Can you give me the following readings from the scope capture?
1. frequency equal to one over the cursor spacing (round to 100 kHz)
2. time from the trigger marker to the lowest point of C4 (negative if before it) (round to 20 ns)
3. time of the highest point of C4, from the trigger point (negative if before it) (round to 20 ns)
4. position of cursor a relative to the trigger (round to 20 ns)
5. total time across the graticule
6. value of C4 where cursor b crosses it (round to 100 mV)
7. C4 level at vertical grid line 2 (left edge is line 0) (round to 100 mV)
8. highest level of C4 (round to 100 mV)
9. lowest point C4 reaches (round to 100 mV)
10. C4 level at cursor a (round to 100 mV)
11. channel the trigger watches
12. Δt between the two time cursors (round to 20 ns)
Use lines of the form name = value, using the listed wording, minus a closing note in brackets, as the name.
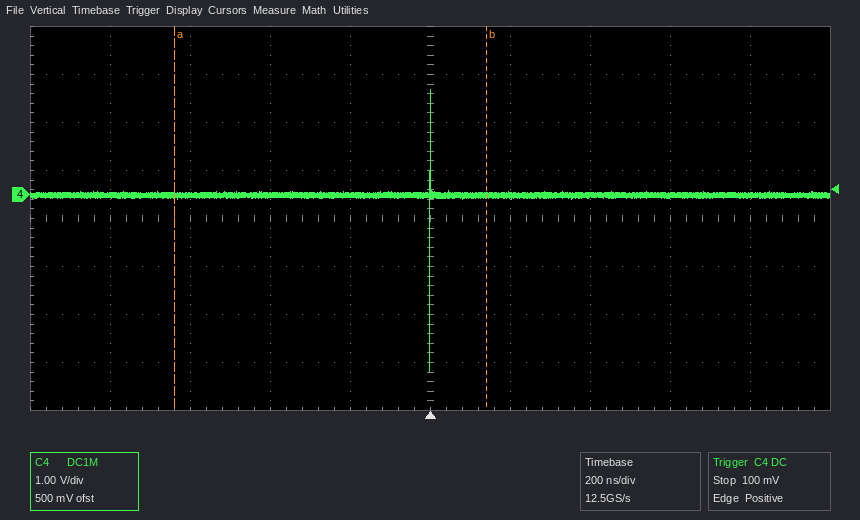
frequency equal to one over the cursor spacing = 1.3 MHz
time from the trigger marker to the lowest point of C4 (negative if before it) = 0 ns
time of the highest point of C4, from the trigger point (negative if before it) = 0 ns
position of cursor a relative to the trigger = -640 ns
total time across the graticule = 2 µs
value of C4 where cursor b crosses it = 0.0 V
C4 level at vertical grid line 2 (left edge is line 0) = 0.0 V
highest level of C4 = 2.2 V
lowest point C4 reaches = -3.7 V
C4 level at cursor a = 0.0 V
channel the trigger watches = C4
Δt between the two time cursors = 780 ns
